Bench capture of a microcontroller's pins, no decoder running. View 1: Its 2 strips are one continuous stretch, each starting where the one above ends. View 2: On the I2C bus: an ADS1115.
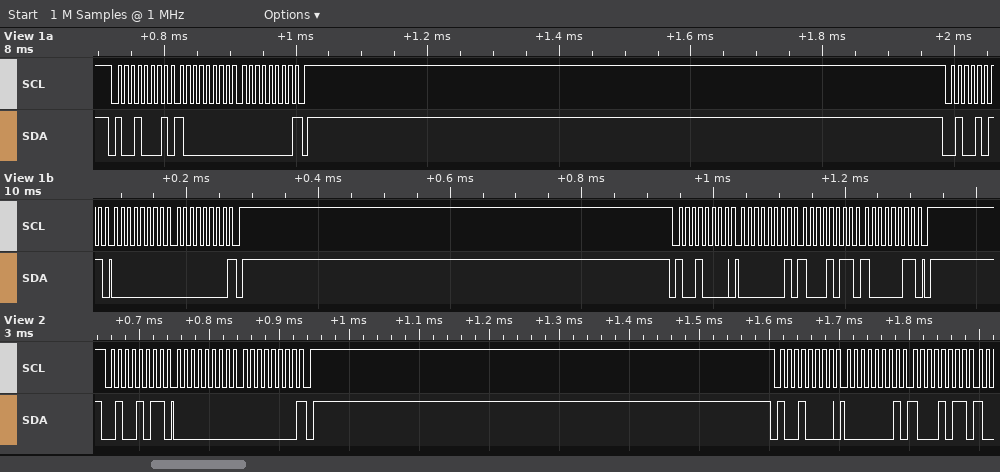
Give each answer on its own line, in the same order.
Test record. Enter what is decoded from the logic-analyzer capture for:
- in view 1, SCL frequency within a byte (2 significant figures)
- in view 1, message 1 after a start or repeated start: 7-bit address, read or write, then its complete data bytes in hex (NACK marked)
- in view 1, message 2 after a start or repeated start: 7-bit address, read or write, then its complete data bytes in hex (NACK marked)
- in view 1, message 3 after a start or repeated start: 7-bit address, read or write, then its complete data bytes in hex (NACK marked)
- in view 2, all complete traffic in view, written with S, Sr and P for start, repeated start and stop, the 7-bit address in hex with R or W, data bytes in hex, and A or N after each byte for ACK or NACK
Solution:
100 kHz
0x48 read: 80 00 NACK
0x25 read: 00 00 NACK
0x48 write: 01 8B 83
S 25R A 00 A 00 N P S 48W A 01 A 8B A
